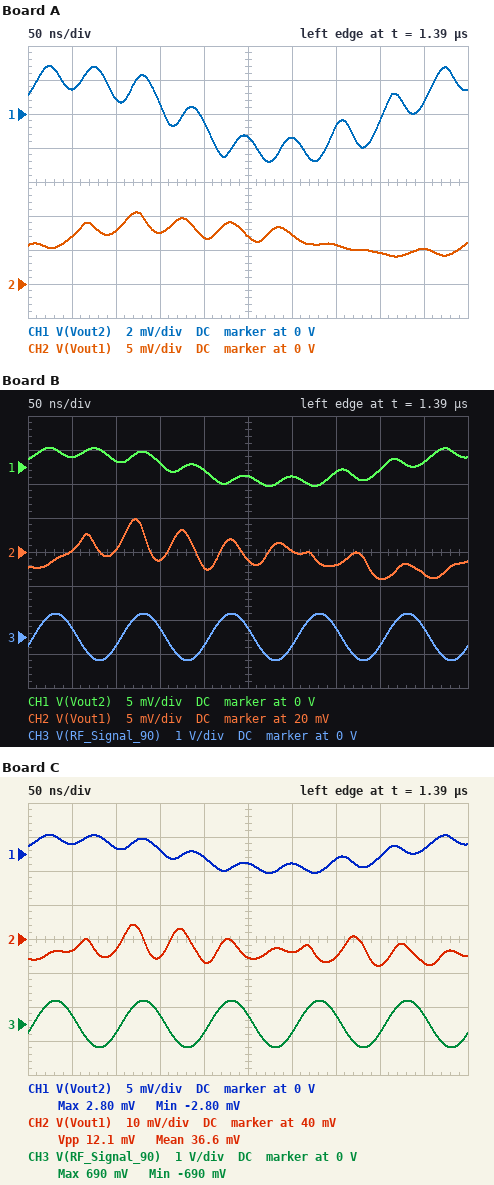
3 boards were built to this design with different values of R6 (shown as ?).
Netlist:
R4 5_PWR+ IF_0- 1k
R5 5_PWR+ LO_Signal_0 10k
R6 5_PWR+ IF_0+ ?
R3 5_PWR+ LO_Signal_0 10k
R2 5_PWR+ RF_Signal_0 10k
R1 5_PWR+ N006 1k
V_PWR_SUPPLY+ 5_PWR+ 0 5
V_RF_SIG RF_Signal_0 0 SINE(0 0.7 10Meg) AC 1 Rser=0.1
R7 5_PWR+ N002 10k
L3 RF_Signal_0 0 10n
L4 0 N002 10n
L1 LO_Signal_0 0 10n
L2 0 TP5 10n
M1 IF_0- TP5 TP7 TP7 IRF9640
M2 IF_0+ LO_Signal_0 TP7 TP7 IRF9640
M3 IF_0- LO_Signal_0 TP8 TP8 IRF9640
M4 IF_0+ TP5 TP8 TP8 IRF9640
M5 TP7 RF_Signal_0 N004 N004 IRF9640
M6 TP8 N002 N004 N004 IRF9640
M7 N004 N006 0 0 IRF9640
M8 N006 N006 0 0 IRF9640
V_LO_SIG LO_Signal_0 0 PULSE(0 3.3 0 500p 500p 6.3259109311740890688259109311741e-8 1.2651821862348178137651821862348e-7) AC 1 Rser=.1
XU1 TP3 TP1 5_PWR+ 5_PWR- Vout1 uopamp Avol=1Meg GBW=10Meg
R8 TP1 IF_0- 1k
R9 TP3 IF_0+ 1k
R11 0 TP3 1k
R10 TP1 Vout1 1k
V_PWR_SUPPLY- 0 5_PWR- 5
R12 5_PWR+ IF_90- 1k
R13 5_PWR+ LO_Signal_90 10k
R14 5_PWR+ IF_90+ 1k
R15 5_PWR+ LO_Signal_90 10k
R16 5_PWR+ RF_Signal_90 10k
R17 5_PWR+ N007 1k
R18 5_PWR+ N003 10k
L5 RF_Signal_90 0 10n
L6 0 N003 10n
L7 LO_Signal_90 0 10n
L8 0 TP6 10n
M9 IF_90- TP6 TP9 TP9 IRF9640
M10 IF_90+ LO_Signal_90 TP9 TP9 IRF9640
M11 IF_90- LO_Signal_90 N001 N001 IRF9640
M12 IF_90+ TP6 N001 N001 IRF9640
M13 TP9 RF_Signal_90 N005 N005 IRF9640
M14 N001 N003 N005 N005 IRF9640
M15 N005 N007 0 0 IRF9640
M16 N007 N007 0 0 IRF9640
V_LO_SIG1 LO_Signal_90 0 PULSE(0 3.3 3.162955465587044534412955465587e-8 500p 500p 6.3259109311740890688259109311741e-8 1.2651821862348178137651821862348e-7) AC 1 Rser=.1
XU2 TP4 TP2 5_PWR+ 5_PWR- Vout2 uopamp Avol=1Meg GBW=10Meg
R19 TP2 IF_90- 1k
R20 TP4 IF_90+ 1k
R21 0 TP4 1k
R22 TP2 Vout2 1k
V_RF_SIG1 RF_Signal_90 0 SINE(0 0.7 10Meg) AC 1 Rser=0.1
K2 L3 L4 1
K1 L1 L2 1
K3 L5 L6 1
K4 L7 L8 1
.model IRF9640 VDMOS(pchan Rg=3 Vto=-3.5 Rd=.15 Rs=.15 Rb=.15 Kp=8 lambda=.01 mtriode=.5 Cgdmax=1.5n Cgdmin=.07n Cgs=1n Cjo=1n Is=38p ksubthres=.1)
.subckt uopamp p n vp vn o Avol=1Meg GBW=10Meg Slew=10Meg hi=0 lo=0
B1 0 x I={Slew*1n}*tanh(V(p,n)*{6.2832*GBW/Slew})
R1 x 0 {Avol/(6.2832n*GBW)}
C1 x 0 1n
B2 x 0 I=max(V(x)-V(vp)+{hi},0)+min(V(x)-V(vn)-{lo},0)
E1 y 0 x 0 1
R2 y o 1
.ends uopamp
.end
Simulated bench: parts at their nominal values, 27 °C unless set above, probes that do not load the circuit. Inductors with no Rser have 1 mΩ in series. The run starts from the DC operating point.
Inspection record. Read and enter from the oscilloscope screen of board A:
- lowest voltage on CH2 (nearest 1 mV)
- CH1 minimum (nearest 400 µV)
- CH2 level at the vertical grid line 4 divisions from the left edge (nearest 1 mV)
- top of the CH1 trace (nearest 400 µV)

4 mV
-2.8 mV
7 mV
2.8 mV
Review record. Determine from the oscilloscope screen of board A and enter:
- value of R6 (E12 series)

820 Ω
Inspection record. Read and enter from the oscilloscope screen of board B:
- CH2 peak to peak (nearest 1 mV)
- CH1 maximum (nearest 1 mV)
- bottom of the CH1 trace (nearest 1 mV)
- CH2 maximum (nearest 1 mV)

9 mV
3 mV
-3 mV
25 mV
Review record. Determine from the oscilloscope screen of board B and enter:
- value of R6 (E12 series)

560 Ω
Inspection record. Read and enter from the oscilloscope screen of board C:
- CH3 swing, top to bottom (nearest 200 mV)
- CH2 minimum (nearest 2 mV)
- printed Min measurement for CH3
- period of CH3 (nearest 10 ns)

1.4 V
32 mV
-690 mV
100 ns
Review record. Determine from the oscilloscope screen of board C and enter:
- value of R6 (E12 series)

330 Ω
